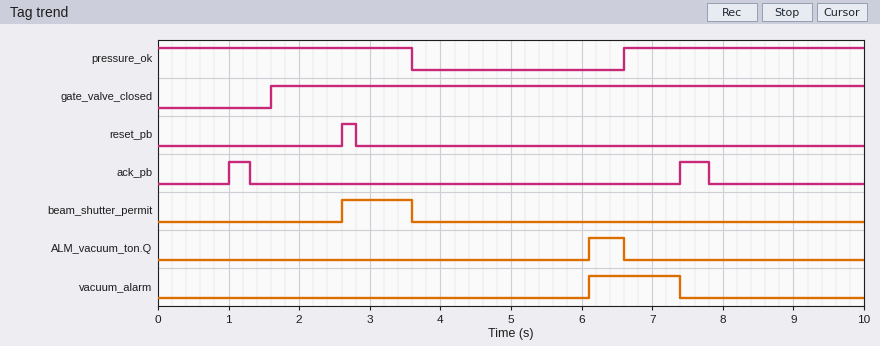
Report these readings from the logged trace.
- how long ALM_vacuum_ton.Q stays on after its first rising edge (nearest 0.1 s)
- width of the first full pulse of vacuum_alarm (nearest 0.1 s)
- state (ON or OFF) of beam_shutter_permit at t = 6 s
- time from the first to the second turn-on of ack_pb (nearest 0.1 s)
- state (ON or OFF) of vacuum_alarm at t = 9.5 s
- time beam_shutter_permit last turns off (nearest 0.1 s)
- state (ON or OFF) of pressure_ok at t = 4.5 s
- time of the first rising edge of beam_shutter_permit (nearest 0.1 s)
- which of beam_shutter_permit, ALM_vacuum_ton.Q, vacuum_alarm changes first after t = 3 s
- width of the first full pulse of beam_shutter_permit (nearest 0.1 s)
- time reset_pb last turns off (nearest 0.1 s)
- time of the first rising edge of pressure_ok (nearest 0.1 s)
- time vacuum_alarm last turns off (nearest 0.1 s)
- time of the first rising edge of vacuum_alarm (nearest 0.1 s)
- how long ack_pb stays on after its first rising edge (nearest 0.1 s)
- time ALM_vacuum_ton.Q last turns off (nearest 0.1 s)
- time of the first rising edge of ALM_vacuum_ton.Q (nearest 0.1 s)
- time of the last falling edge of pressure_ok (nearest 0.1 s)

0.5 s
1.3 s
OFF
6.4 s
OFF
3.6 s
OFF
2.6 s
beam_shutter_permit
1.0 s
2.8 s
6.6 s
7.4 s
6.1 s
0.3 s
6.6 s
6.1 s
3.6 s
